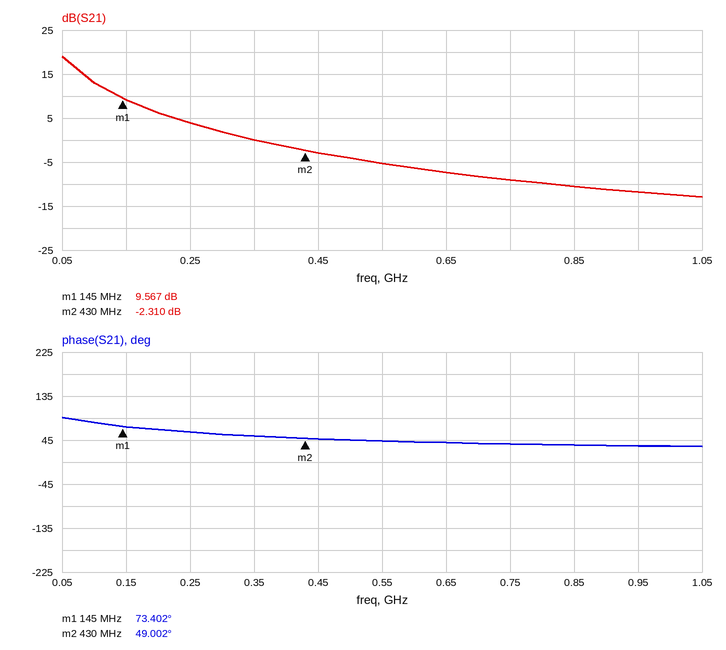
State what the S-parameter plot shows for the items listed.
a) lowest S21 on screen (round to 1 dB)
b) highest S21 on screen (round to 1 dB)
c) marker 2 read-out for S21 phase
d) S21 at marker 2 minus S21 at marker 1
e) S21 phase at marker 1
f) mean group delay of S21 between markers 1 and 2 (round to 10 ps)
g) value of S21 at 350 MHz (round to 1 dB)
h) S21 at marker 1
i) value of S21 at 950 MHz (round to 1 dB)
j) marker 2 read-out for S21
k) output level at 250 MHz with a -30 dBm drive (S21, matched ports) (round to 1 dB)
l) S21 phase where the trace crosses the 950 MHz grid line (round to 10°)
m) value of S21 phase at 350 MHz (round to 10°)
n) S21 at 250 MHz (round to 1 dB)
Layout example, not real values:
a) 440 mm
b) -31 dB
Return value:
a) -13 dB
b) 19 dB
c) 49.002°
d) -11.877 dB
e) 73.402°
f) 240 ps
g) 0 dB
h) 9.567 dB
i) -12 dB
j) -2.310 dB
k) -26 dBm
l) 30°
m) 50°
n) 4 dB
